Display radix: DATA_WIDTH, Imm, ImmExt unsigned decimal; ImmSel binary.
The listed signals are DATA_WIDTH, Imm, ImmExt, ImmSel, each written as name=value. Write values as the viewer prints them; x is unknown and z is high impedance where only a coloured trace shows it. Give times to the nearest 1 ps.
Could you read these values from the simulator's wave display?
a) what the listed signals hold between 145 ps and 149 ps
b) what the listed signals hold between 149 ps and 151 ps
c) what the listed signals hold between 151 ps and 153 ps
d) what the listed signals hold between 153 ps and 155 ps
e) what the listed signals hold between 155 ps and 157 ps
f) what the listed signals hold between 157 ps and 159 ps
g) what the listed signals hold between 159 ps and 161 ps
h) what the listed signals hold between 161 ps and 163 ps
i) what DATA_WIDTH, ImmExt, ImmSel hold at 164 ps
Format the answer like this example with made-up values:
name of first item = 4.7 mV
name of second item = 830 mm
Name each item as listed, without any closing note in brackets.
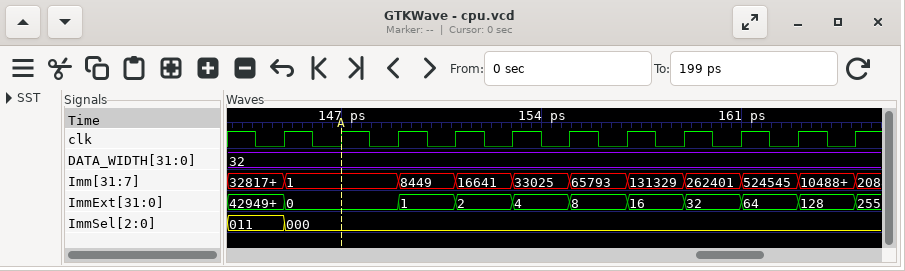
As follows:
what the listed signals hold between 145 ps and 149 ps = DATA_WIDTH=32, Imm=1, ImmExt=0, ImmSel=000
what the listed signals hold between 149 ps and 151 ps = DATA_WIDTH=32, Imm=8449, ImmExt=1, ImmSel=000
what the listed signals hold between 151 ps and 153 ps = DATA_WIDTH=32, Imm=16641, ImmExt=2, ImmSel=000
what the listed signals hold between 153 ps and 155 ps = DATA_WIDTH=32, Imm=33025, ImmExt=4, ImmSel=000
what the listed signals hold between 155 ps and 157 ps = DATA_WIDTH=32, Imm=65793, ImmExt=8, ImmSel=000
what the listed signals hold between 157 ps and 159 ps = DATA_WIDTH=32, Imm=131329, ImmExt=16, ImmSel=000
what the listed signals hold between 159 ps and 161 ps = DATA_WIDTH=32, Imm=262401, ImmExt=32, ImmSel=000
what the listed signals hold between 161 ps and 163 ps = DATA_WIDTH=32, Imm=524545, ImmExt=64, ImmSel=000
what DATA_WIDTH, ImmExt, ImmSel hold at 164 ps = DATA_WIDTH=32, ImmExt=128, ImmSel=000
